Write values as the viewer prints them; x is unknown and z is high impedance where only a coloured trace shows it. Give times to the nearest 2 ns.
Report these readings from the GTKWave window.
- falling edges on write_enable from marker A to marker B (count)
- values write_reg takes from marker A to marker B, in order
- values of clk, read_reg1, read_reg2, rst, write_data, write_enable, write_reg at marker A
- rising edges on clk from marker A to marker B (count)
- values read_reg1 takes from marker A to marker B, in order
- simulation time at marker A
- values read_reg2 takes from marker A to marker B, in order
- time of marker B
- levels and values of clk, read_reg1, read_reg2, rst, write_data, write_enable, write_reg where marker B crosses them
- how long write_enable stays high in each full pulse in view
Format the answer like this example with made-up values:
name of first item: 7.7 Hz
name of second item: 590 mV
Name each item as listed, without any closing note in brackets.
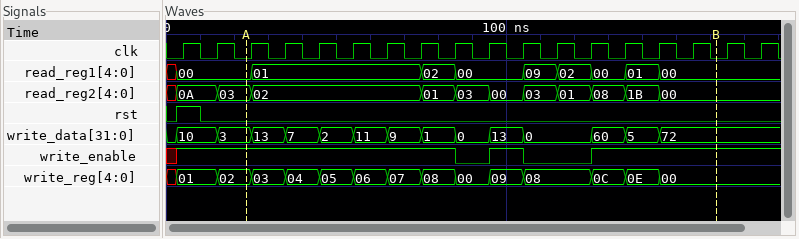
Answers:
falling edges on write_enable from marker A to marker B: 2
values write_reg takes from marker A to marker B, in order: 02, 03, 04, 05, 06, 07, 08, 00, 09, 08, 0C, 0E, 00
values of clk, read_reg1, read_reg2, rst, write_data, write_enable, write_reg at marker A: clk=0, read_reg1=00, read_reg2=03, rst=0, write_data=3, write_enable=1, write_reg=02
rising edges on clk from marker A to marker B: 14
values read_reg1 takes from marker A to marker B, in order: 00, 01, 02, 00, 09, 02, 00, 01, 00
simulation time at marker A: 24 ns
values read_reg2 takes from marker A to marker B, in order: 03, 02, 01, 03, 00, 03, 01, 08, 1B, 00
time of marker B: 162 ns
levels and values of clk, read_reg1, read_reg2, rst, write_data, write_enable, write_reg where marker B crosses them: clk=0, read_reg1=00, read_reg2=00, rst=0, write_data=72, write_enable=1, write_reg=00
how long write_enable stays high in each full pulse in view: 10 ns
